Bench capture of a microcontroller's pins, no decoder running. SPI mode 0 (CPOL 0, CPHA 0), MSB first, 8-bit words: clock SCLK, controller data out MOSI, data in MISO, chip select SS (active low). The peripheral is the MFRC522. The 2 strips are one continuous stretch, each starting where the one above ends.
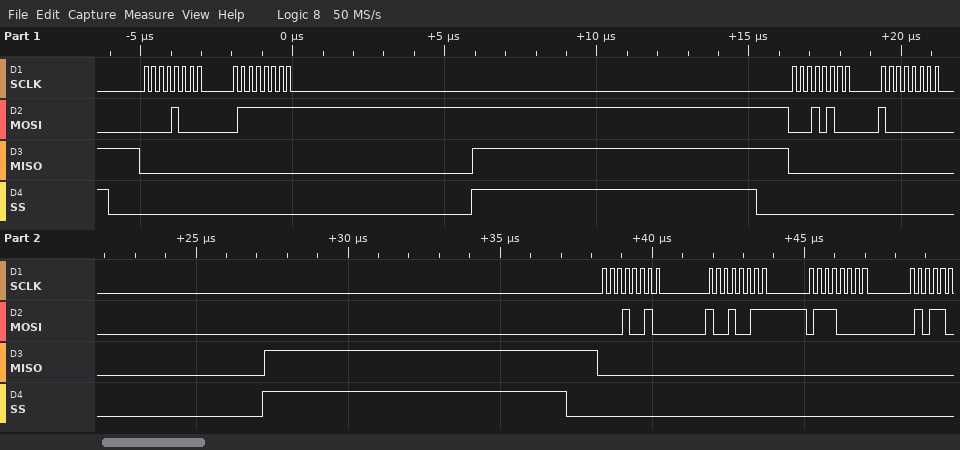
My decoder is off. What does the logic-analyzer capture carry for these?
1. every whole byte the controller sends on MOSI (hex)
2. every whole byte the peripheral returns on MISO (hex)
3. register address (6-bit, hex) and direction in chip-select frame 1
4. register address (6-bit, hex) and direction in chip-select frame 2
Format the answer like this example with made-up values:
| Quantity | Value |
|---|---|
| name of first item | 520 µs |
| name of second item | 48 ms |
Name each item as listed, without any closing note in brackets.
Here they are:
| Quantity | Value |
|---|---|
| every whole byte the controller sends on MOSI | 0x08 0x7F 0x14 0x80 0x12 0x93 0x70 |
| every whole byte the peripheral returns on MISO | 0x00 0x00 0x00 0x00 0x00 0x00 0x00 |
| register address (6-bit, hex) and direction in chip-select frame 1 | 0x04 write |
| register address (6-bit, hex) and direction in chip-select frame 2 | 0x0A write |
